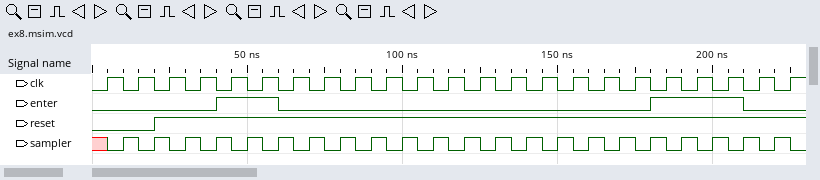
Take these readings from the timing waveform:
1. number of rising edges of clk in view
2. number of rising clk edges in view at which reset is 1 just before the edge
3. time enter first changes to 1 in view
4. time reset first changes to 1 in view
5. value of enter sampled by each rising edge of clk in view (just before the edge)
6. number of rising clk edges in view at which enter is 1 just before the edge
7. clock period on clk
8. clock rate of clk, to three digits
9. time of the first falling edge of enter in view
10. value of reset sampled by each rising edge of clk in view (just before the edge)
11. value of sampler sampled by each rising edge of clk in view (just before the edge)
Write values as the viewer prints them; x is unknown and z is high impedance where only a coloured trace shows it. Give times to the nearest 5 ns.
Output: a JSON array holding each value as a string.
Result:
["23", "21", "40 ns", "20 ns", "0 0 0 0 1 1 0 0 0 0 0 0 0 0 0 0 0 0 1 1 1 0 0", "5", "10 ns", "100 MHz", "60 ns", "0 0 1 1 1 1 1 1 1 1 1 1 1 1 1 1 1 1 1 1 1 1 1", "x 1 1 1 1 1 1 1 1 1 1 1 1 1 1 1 1 1 1 1 1 1 1"]
